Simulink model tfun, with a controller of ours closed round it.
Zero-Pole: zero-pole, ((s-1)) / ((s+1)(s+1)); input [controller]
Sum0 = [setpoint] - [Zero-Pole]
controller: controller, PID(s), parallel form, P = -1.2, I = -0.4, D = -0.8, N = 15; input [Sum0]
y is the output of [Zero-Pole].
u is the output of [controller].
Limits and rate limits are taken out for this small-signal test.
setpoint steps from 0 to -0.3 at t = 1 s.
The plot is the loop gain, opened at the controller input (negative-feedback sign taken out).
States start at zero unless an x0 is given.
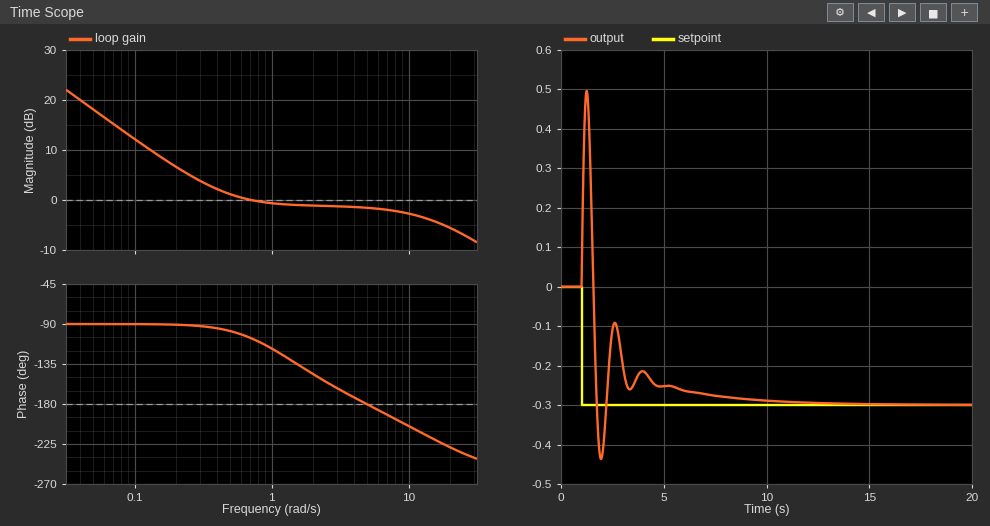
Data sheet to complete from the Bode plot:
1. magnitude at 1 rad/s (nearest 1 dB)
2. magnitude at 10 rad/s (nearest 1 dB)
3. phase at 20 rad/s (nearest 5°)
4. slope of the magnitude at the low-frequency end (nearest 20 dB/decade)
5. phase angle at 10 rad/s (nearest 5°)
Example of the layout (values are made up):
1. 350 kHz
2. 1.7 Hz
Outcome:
1. -1 dB
2. -3 dB
3. -230°
4. -20 dB/decade
5. -205°
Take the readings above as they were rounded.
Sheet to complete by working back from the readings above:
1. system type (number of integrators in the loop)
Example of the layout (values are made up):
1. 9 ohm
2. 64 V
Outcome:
1. 1
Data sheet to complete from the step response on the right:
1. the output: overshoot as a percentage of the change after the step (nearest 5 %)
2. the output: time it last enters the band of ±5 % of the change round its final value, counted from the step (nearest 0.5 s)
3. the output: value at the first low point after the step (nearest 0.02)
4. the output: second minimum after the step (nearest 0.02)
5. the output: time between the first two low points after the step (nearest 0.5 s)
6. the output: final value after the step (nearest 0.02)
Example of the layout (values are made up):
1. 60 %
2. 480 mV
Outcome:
1. 45 %
2. 8.0 s
3. -0.44
4. -0.26
5. 1.5 s
6. -0.30
